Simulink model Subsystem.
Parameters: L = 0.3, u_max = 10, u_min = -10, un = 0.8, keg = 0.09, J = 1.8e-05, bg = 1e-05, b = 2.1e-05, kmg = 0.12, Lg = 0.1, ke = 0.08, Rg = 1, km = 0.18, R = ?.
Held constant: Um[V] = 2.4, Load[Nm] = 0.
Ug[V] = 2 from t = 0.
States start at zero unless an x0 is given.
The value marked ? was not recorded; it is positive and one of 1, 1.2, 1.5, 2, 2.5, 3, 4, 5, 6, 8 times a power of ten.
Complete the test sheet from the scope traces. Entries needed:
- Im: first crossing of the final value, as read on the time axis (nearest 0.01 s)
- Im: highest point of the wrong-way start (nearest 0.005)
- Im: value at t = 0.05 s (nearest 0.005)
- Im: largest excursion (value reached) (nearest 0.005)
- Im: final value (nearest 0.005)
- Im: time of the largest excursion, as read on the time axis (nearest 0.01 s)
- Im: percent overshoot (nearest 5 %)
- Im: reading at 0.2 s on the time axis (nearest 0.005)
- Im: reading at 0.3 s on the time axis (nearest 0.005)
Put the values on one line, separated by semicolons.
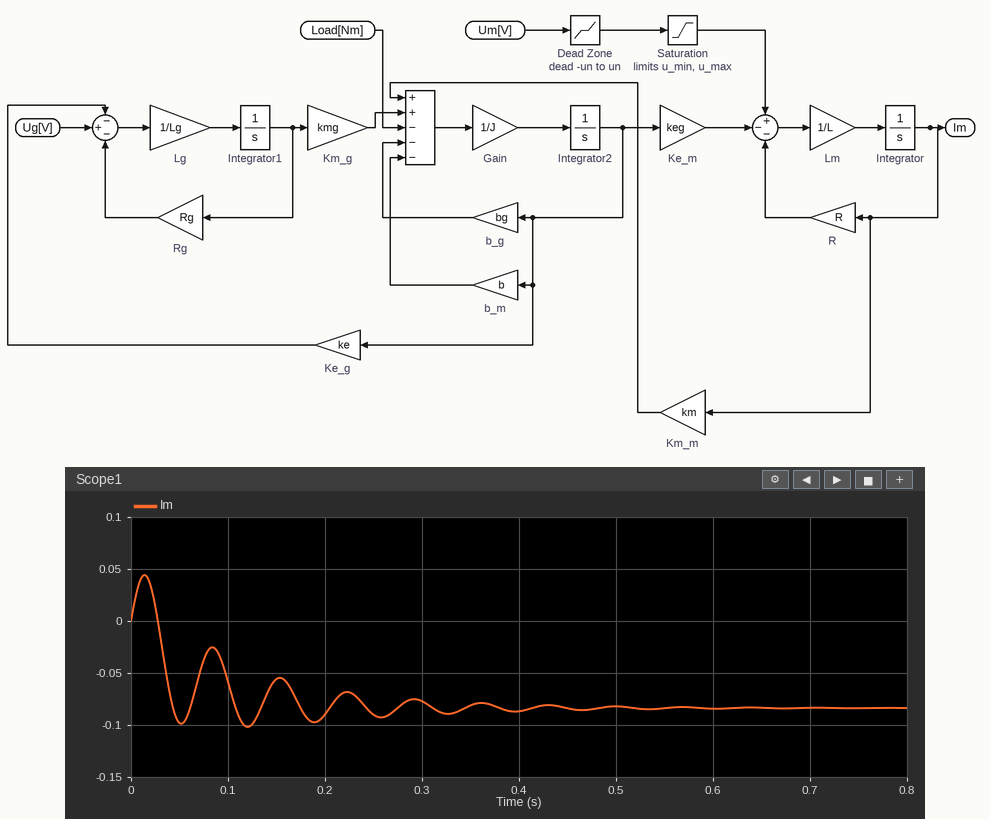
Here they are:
0.04 s; 0.045; -0.100; -0.100; -0.085; 0.12 s; 20 %; -0.090; -0.075
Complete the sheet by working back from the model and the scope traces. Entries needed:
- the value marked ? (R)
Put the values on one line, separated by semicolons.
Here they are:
6
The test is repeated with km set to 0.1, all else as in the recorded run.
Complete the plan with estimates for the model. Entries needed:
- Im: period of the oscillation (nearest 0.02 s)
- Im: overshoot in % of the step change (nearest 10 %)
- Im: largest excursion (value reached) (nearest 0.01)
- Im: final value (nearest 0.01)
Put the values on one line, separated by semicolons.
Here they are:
0.08 s; 30 %; -0.12; -0.09
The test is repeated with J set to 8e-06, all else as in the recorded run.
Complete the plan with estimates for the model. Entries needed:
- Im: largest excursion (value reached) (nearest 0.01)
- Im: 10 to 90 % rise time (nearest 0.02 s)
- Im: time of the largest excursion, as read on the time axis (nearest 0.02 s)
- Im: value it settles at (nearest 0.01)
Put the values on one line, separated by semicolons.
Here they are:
-0.09; 0.06 s; 0.18 s; -0.08
